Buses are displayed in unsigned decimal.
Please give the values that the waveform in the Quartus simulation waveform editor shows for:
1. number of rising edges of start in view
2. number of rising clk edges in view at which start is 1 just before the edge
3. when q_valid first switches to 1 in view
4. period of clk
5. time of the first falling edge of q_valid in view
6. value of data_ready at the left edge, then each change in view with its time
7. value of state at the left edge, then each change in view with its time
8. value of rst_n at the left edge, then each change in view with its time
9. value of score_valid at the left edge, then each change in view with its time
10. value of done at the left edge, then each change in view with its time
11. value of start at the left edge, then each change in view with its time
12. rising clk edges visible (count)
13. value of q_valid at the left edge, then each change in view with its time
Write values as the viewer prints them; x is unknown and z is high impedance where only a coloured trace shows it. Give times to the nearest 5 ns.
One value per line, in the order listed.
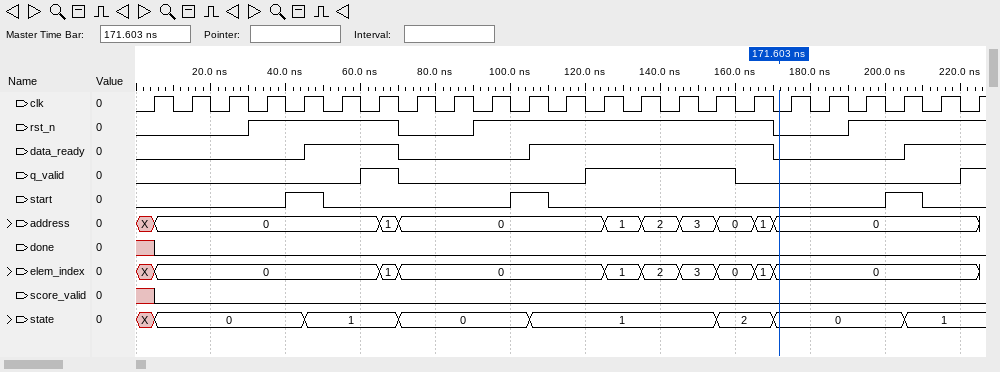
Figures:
3
3
60 ns
10 ns
70 ns
0, 1 at 45 ns, 0 at 70 ns, 1 at 105 ns, 0 at 170 ns, 1 at 205 ns
X, 0 at 5 ns, 1 at 45 ns, 0 at 70 ns, 1 at 105 ns, 2 at 155 ns, 0 at 170 ns, 1 at 205 ns
0, 1 at 30 ns, 0 at 70 ns, 1 at 90 ns, 0 at 170 ns, 1 at 190 ns
x, 0 at 5 ns
x, 0 at 5 ns
0, 1 at 40 ns, 0 at 50 ns, 1 at 100 ns, 0 at 110 ns, 1 at 200 ns, 0 at 210 ns
23
0, 1 at 60 ns, 0 at 70 ns, 1 at 120 ns, 0 at 160 ns, 1 at 220 ns
